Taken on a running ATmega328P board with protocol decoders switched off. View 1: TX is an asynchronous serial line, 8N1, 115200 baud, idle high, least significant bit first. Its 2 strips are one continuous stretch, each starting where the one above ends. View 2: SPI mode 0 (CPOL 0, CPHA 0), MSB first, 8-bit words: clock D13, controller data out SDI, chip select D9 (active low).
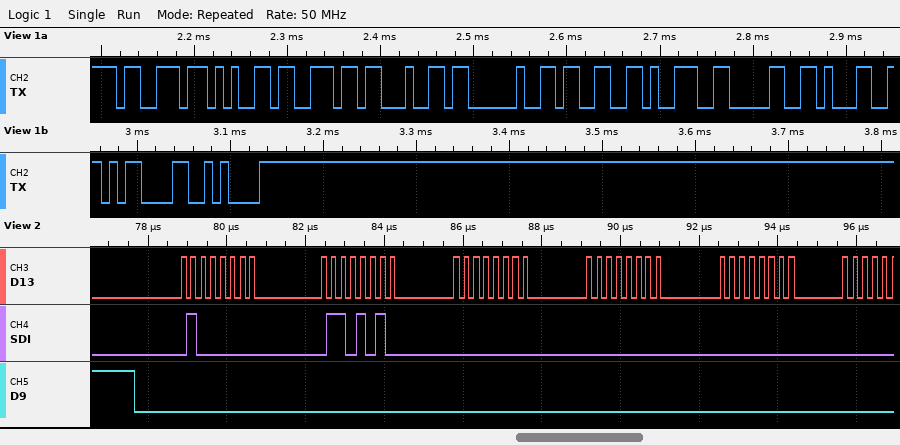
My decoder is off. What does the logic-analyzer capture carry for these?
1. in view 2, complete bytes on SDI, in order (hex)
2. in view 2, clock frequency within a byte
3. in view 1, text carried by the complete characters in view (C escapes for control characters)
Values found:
40 6A 00 00 00
4 MHz
"send 3901\r\n"
